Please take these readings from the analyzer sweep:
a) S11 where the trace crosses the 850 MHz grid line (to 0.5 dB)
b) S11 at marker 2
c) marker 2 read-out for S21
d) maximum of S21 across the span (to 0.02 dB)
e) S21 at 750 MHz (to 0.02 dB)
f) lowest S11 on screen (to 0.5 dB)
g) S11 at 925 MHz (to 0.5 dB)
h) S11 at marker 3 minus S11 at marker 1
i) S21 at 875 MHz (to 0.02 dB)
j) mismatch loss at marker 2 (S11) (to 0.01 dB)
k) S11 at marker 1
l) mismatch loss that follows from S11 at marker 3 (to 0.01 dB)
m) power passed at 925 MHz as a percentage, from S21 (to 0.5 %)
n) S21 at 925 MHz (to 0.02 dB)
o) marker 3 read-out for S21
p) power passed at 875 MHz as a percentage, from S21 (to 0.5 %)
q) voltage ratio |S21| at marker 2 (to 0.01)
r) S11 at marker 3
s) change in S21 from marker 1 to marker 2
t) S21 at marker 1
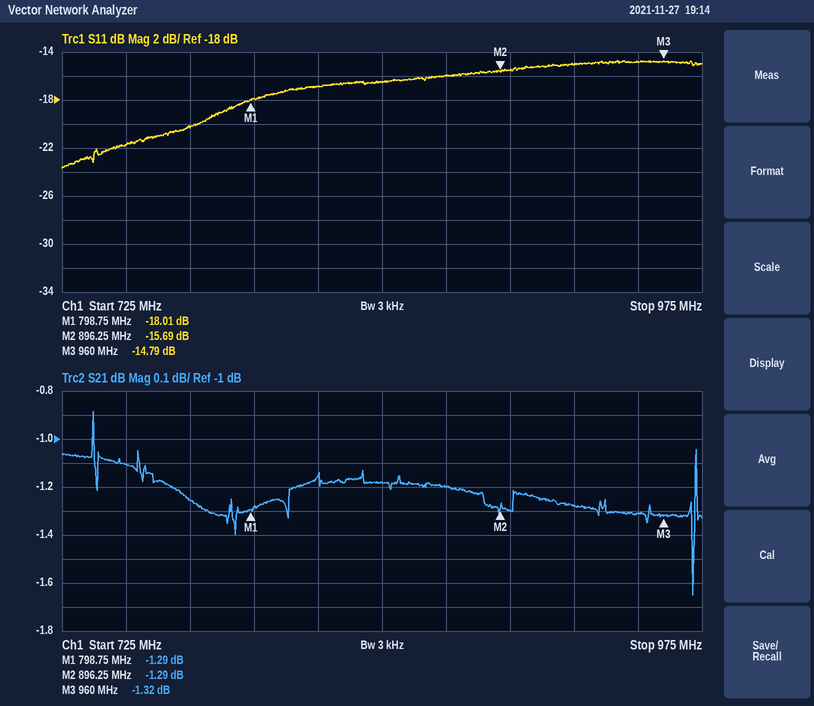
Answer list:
-16.5 dB
-15.69 dB
-1.29 dB
-0.88 dB
-1.10 dB
-23.5 dB
-15.0 dB
3.22 dB
-1.20 dB
0.12 dB
-18.01 dB
0.15 dB
74.5 %
-1.28 dB
-1.32 dB
76.0 %
0.86
-14.79 dB
0.00 dB
-1.29 dB
